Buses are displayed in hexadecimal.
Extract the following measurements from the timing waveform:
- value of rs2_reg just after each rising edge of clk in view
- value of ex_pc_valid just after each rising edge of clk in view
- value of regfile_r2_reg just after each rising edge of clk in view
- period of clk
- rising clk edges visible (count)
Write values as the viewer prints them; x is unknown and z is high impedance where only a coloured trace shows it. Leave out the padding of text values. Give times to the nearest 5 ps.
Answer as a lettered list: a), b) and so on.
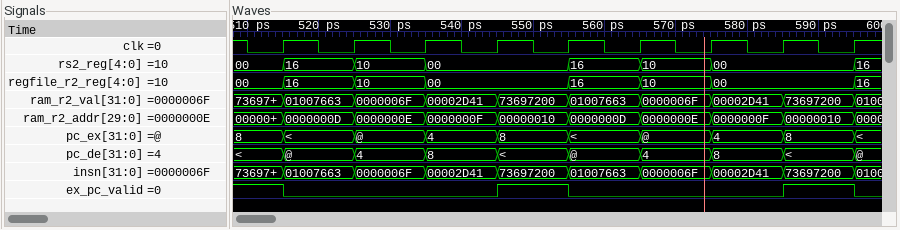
a) 16, 10, 00, 00, 16, 10, 00, 00, 16
b) 0 0 0 1 0 0 0 1 0
c) 16, 10, 00, 00, 16, 10, 00, 00, 16
d) 10 ps
e) 9
